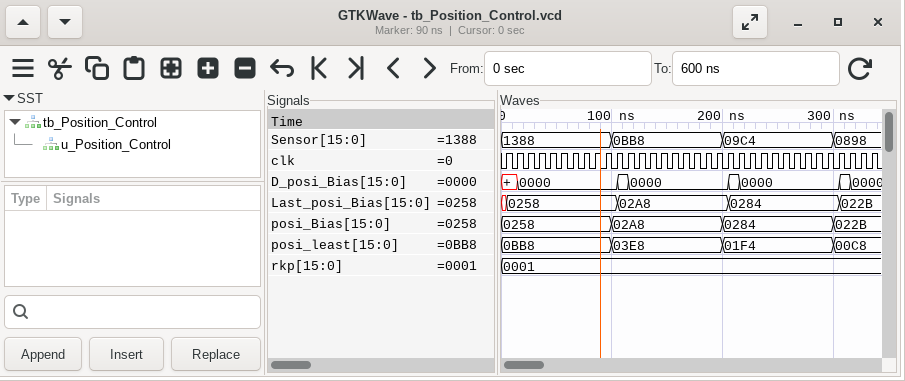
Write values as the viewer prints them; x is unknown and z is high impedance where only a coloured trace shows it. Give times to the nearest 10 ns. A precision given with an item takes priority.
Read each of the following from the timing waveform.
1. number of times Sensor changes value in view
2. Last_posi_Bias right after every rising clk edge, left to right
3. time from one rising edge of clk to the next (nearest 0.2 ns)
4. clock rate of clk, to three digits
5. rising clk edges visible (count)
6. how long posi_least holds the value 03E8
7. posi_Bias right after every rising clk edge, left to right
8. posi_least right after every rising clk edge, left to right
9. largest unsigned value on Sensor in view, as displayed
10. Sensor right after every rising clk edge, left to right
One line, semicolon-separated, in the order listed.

3; 0258, 0258, 0258, 0258, 0258, 0258, 0258, 0258, 0258, 0258, 02A8, 02A8, 02A8, 02A8, 02A8, 02A8, 02A8, 02A8, 02A8, 02A8, 0284, 0284, 0284, 0284, 0284, 0284, 0284, 0284, 0284, 0284, 022B, 022B, 022B, 022B; 10 ns; 100 MHz; 34; 100 ns; 0258, 0258, 0258, 0258, 0258, 0258, 0258, 0258, 0258, 0258, 02A8, 02A8, 02A8, 02A8, 02A8, 02A8, 02A8, 02A8, 02A8, 02A8, 0284, 0284, 0284, 0284, 0284, 0284, 0284, 0284, 0284, 0284, 022B, 022B, 022B, 022B; 0BB8, 0BB8, 0BB8, 0BB8, 0BB8, 0BB8, 0BB8, 0BB8, 0BB8, 0BB8, 03E8, 03E8, 03E8, 03E8, 03E8, 03E8, 03E8, 03E8, 03E8, 03E8, 01F4, 01F4, 01F4, 01F4, 01F4, 01F4, 01F4, 01F4, 01F4, 01F4, 00C8, 00C8, 00C8, 00C8; 1388; 1388, 1388, 1388, 1388, 1388, 1388, 1388, 1388, 1388, 1388, 0BB8, 0BB8, 0BB8, 0BB8, 0BB8, 0BB8, 0BB8, 0BB8, 0BB8, 0BB8, 09C4, 09C4, 09C4, 09C4, 09C4, 09C4, 09C4, 09C4, 09C4, 09C4, 0898, 0898, 0898, 0898
